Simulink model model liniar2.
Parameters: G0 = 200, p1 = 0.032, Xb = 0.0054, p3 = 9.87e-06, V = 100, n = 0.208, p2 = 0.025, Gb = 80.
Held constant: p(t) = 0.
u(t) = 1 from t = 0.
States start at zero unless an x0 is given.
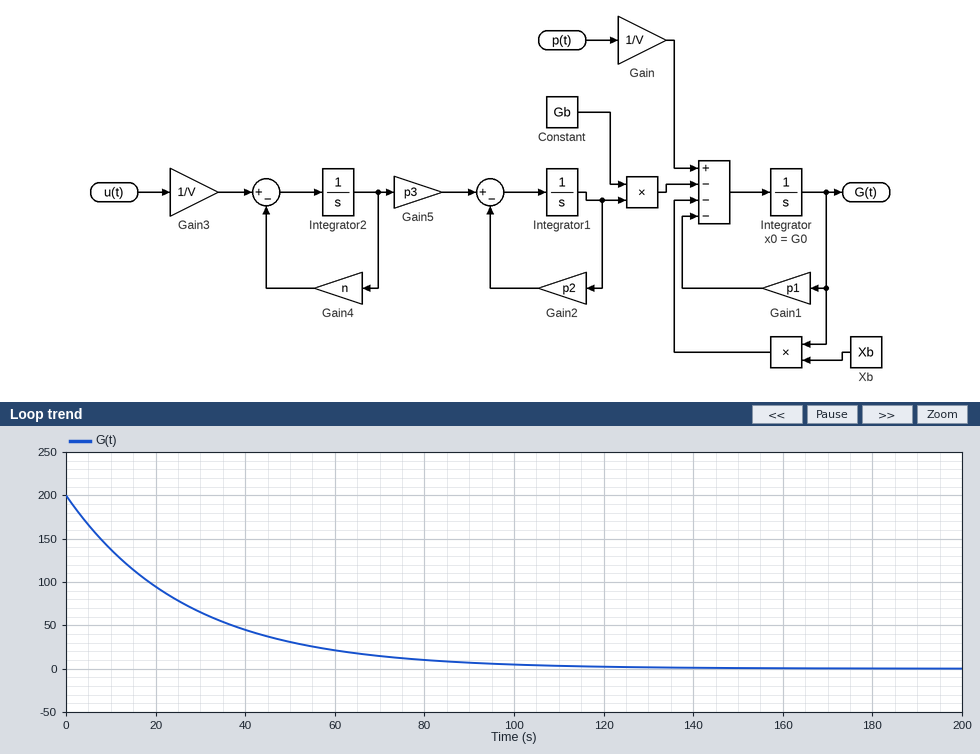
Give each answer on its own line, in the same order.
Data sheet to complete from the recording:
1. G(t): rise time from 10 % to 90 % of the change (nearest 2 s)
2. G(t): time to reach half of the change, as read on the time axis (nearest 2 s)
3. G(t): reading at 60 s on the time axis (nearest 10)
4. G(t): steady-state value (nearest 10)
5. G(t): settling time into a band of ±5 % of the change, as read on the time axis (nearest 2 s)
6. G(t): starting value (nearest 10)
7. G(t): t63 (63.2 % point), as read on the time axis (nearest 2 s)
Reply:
58 s
18 s
20
0
80 s
200
26 s
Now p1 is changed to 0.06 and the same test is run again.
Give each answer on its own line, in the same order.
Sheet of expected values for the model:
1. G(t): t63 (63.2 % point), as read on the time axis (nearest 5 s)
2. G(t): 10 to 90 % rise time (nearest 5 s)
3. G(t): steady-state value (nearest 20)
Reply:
15 s
35 s
0
